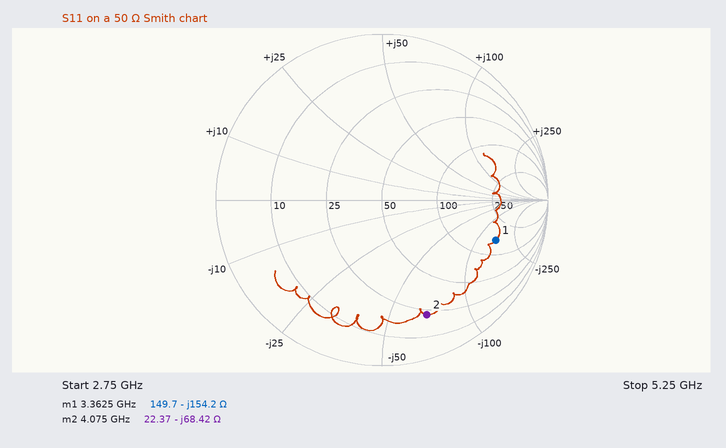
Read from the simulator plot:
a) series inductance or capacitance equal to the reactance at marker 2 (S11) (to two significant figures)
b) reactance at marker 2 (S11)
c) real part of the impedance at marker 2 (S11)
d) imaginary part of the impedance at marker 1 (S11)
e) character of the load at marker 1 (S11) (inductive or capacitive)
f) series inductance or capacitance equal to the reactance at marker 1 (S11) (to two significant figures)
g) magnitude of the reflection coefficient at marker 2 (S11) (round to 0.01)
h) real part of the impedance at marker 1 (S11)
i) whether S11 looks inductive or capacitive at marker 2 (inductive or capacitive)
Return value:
570 fF
-68.42 Ω
22.37 Ω
-154.2 Ω
capacitive
310 fF
0.74
149.7 Ω
capacitive
